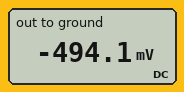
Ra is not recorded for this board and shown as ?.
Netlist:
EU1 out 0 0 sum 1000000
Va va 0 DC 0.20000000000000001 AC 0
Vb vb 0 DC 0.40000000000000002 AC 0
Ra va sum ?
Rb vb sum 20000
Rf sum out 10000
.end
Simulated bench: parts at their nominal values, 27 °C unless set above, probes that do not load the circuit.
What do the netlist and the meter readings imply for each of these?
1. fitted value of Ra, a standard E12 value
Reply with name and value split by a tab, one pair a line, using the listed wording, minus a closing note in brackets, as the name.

fitted value of Ra, a standard E12 value	6.8 kΩ
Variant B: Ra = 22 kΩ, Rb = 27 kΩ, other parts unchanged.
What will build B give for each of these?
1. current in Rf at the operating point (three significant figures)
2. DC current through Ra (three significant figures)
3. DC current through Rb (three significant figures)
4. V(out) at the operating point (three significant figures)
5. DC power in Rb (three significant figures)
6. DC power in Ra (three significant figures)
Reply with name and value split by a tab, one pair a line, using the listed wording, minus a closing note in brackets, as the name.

current in Rf at the operating point	23.9 µA
DC current through Ra	9.09 µA
DC current through Rb	14.8 µA
V(out) at the operating point	-239 mV
DC power in Rb	5.93 µW
DC power in Ra	1.82 µW
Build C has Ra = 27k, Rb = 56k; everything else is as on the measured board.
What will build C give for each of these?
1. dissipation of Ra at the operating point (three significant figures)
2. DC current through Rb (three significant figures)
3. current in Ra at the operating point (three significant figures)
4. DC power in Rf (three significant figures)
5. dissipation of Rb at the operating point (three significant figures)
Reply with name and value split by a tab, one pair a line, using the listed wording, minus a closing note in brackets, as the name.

dissipation of Ra at the operating point	1.48 µW
DC current through Rb	7.14 µA
current in Ra at the operating point	7.41 µA
DC power in Rf	2.12 µW
dissipation of Rb at the operating point	2.86 µW
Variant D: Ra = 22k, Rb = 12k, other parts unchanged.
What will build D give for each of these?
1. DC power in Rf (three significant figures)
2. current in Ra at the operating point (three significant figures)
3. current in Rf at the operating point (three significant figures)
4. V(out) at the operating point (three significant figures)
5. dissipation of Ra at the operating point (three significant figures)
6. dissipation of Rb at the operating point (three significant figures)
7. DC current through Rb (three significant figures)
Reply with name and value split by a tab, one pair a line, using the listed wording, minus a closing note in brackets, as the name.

DC power in Rf	18.0 µW
current in Ra at the operating point	9.09 µA
current in Rf at the operating point	42.4 µA
V(out) at the operating point	-424 mV
dissipation of Ra at the operating point	1.82 µW
dissipation of Rb at the operating point	13.3 µW
DC current through Rb	33.3 µA
